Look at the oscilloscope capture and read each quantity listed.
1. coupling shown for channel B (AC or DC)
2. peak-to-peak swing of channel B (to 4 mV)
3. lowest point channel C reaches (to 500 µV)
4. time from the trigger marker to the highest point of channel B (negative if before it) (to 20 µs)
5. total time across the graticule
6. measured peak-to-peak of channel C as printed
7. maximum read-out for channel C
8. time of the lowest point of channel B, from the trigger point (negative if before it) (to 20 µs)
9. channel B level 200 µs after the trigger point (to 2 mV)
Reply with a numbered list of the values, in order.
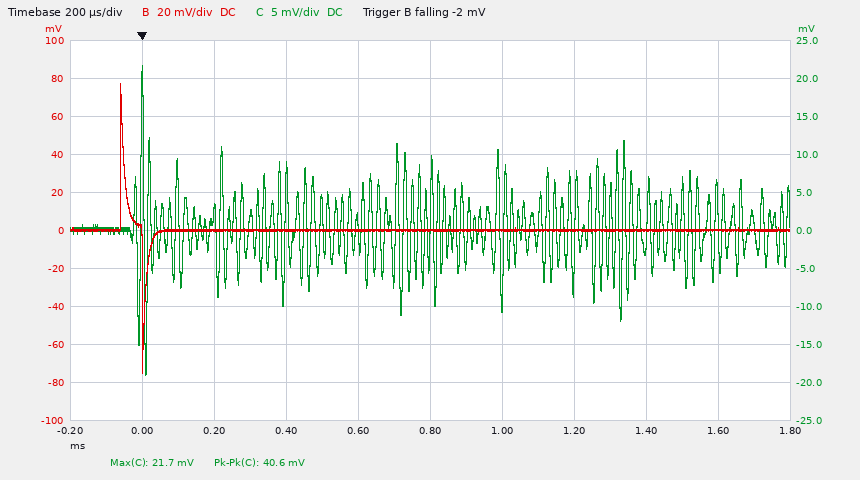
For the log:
1. DC
2. 152 mV
3. -19.0 mV
4. -60 µs
5. 2 ms
6. 40.6 mV
7. 21.7 mV
8. 0 µs
9. 0 mV
